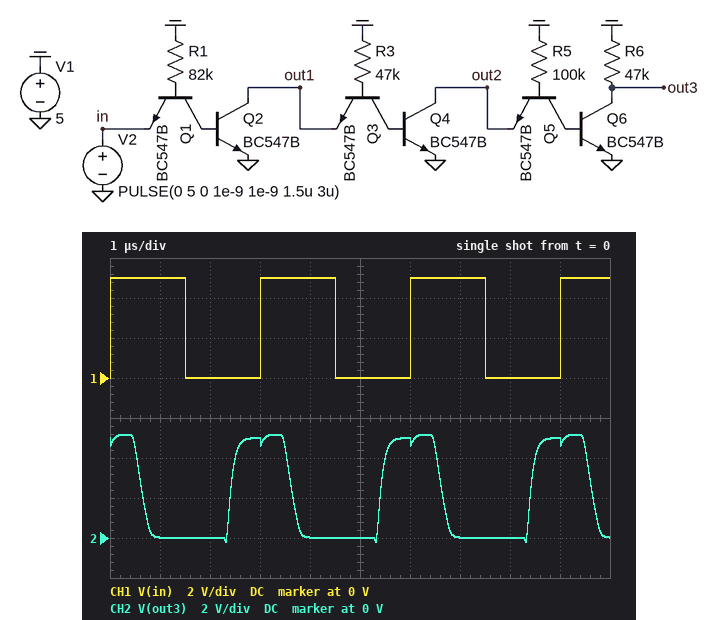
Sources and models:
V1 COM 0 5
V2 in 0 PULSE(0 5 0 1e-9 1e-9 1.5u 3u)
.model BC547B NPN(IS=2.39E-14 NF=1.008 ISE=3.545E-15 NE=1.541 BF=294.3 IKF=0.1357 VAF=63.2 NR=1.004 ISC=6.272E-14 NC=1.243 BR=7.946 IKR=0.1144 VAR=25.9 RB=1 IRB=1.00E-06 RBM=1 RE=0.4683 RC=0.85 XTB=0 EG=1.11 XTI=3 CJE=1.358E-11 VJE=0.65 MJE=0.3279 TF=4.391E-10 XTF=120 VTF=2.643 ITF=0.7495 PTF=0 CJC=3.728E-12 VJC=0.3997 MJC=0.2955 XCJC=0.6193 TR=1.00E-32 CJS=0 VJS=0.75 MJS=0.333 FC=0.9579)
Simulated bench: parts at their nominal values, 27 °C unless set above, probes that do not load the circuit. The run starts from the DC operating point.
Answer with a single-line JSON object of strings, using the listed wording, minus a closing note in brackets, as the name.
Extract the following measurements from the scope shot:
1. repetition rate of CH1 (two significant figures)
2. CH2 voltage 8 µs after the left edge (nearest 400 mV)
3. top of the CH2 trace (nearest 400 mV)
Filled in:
{"repetition rate of CH1": "330 kHz", "CH2 voltage 8 µs after the left edge": "0 V", "top of the CH2 trace": "5.2 V"}
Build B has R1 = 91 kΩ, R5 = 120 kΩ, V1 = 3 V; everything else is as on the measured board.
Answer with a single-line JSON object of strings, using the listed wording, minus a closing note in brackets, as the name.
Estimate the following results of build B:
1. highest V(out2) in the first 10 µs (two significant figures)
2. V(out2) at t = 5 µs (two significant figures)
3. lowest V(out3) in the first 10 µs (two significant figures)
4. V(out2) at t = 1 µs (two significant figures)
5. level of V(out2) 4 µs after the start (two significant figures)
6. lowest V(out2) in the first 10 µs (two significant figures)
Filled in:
{"highest V(out2) in the first 10 µs": "600 mV", "V(out2) at t = 5 µs": "590 mV", "lowest V(out3) in the first 10 µs": "-110 mV", "V(out2) at t = 1 µs": "510 mV", "level of V(out2) 4 µs after the start": "570 mV", "lowest V(out2) in the first 10 µs": "-400 mV"}
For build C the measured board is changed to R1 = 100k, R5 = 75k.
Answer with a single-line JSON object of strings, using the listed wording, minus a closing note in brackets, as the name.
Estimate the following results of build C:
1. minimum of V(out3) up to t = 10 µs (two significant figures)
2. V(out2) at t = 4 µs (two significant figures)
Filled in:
{"minimum of V(out3) up to t = 10 µs": "-230 mV", "V(out2) at t = 4 µs": "620 mV"}
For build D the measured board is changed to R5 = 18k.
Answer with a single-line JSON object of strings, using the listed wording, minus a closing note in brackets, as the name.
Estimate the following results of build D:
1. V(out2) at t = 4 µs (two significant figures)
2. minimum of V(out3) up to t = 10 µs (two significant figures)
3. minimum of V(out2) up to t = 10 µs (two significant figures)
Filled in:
{"V(out2) at t = 4 µs": "650 mV", "minimum of V(out3) up to t = 10 µs": "-270 mV", "minimum of V(out2) up to t = 10 µs": "-370 mV"}
